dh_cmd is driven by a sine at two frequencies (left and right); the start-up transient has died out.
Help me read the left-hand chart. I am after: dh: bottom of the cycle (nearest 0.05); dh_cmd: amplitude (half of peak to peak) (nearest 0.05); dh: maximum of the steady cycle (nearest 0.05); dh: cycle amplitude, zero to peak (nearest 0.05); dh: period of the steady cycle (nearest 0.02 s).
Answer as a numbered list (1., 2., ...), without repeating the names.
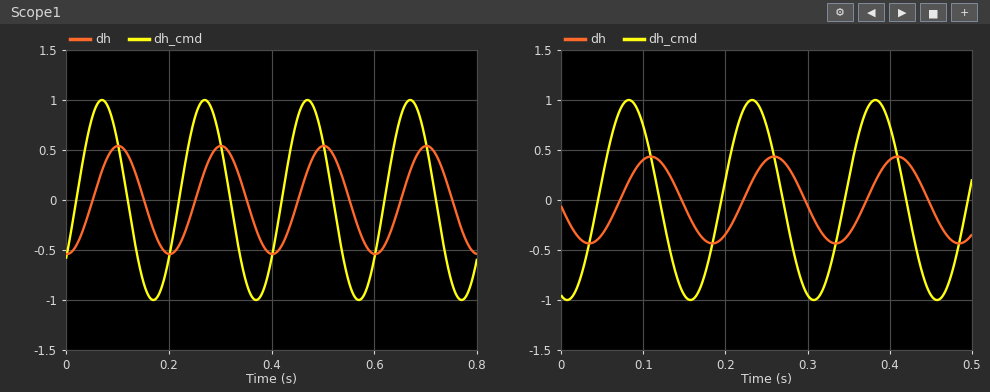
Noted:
1. -0.55
2. 1.00
3. 0.55
4. 0.55
5. 0.20 s
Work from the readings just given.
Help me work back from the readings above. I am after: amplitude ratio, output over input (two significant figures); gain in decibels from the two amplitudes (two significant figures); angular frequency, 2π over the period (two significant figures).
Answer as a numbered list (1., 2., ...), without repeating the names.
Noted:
1. 0.55
2. -5.2 dB
3. 31 rad/s
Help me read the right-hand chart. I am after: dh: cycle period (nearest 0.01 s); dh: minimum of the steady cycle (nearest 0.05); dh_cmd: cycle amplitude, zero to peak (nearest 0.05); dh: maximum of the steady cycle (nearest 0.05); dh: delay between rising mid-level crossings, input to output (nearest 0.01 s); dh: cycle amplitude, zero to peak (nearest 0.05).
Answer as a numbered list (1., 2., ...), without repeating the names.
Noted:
1. 0.15 s
2. -0.45
3. 1.00
4. 0.45
5. 0.03 s
6. 0.45
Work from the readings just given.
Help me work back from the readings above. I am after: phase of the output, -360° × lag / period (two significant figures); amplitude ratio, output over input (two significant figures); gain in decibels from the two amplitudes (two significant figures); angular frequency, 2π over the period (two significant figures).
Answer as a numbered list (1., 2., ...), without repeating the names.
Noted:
1. -72°
2. 0.45
3. -6.9 dB
4. 42 rad/s
